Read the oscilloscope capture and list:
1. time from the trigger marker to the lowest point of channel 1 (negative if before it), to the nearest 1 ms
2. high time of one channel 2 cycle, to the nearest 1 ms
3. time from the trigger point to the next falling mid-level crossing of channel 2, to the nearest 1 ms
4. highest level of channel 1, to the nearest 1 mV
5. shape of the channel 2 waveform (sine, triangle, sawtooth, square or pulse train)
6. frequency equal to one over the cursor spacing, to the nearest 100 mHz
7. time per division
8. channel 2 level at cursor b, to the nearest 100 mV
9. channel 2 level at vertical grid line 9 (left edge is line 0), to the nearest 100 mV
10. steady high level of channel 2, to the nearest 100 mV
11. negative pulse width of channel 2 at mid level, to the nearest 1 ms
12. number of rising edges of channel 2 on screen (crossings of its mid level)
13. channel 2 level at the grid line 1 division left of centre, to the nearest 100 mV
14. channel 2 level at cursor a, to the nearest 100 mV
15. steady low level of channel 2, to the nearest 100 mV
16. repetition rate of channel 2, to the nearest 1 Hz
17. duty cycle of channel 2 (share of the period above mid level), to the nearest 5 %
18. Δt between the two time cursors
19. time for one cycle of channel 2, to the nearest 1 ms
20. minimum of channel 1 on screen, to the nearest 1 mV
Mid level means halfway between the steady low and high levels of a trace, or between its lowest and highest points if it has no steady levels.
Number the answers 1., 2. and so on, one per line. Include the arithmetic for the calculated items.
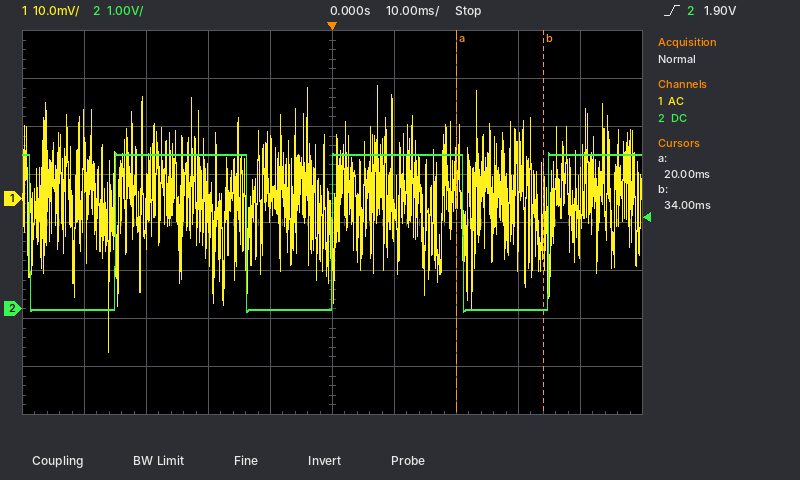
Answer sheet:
1. -36 ms
2. 21 ms
3. 21 ms
4. 24 mV
5. pulse train
6. 1 / 14 ms ≈ 71.4 Hz
7. 10 ms
8. 0.0 V
9. 3.2 V
10. 3.2 V
11. 14 ms
12. 3
13. 0.0 V
14. 3.2 V
15. 0.0 V
16. 1 / 35 ms ≈ 29 Hz
17. 21 ms / 35 ms ≈ 60 %
18. 34 ms − (20 ms) = 14 ms
19. 35 ms
20. -32 mV
